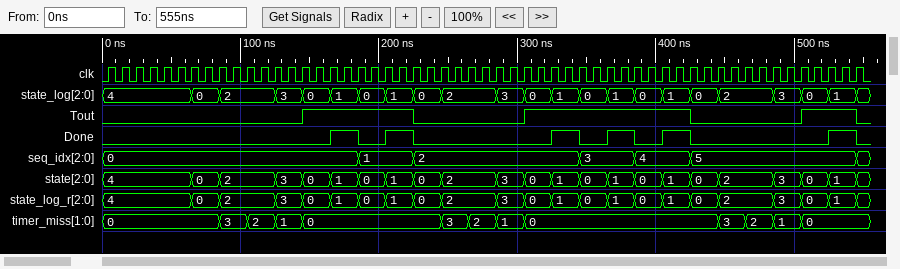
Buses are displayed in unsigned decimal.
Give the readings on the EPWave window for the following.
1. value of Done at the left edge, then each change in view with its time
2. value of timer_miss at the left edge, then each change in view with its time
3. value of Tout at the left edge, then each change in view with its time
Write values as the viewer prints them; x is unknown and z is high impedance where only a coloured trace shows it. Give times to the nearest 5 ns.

0, 1 at 165 ns, 0 at 185 ns, 1 at 205 ns, 0 at 225 ns, 1 at 325 ns, 0 at 345 ns, 1 at 365 ns, 0 at 385 ns, 1 at 405 ns, 0 at 425 ns, 1 at 525 ns, 0 at 545 ns
0, 3 at 85 ns, 2 at 105 ns, 1 at 125 ns, 0 at 145 ns, 3 at 245 ns, 2 at 265 ns, 1 at 285 ns, 0 at 305 ns, 3 at 445 ns, 2 at 465 ns, 1 at 485 ns, 0 at 505 ns
0, 1 at 145 ns, 0 at 225 ns, 1 at 305 ns, 0 at 425 ns, 1 at 505 ns, 0 at 545 ns
